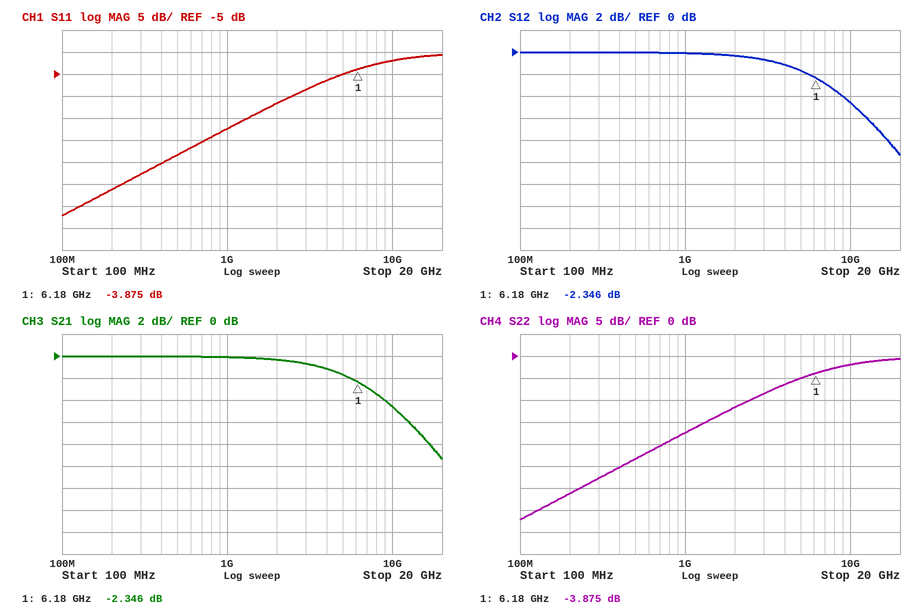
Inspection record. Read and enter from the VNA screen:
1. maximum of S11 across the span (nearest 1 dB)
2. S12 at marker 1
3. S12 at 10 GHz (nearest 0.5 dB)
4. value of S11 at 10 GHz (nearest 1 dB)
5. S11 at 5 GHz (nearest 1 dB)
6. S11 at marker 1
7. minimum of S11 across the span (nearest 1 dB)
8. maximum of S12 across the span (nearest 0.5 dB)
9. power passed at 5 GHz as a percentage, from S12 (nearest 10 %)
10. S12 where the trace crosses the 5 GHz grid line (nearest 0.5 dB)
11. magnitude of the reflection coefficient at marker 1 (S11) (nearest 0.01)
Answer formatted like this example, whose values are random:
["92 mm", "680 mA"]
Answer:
["-1 dB", "-2.346 dB", "-4.5 dB", "-2 dB", "-5 dB", "-3.875 dB", "-37 dB", "0.0 dB", "70 %", "-1.5 dB", "0.64"]
